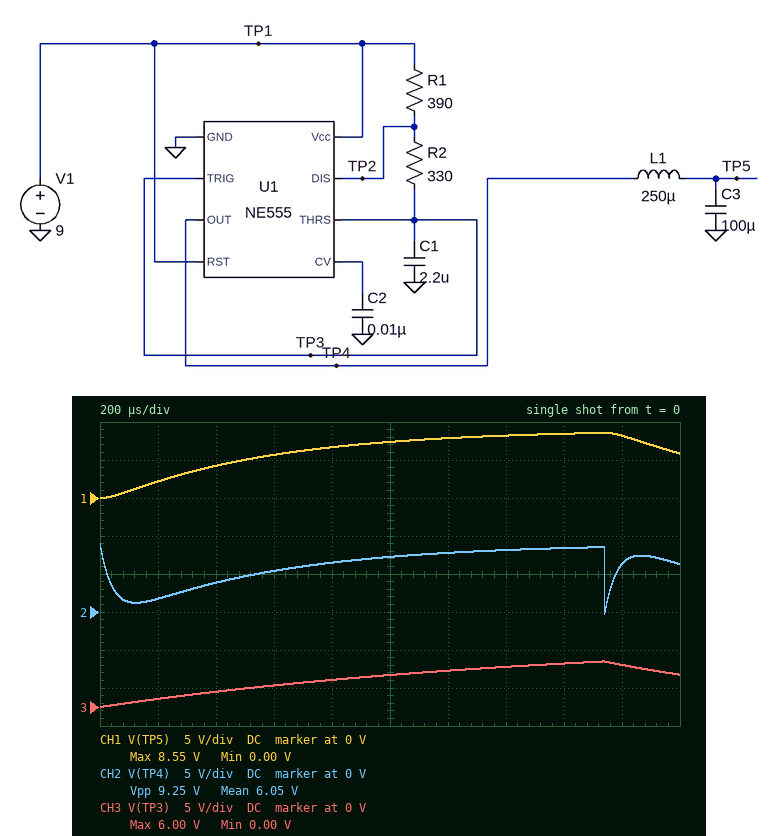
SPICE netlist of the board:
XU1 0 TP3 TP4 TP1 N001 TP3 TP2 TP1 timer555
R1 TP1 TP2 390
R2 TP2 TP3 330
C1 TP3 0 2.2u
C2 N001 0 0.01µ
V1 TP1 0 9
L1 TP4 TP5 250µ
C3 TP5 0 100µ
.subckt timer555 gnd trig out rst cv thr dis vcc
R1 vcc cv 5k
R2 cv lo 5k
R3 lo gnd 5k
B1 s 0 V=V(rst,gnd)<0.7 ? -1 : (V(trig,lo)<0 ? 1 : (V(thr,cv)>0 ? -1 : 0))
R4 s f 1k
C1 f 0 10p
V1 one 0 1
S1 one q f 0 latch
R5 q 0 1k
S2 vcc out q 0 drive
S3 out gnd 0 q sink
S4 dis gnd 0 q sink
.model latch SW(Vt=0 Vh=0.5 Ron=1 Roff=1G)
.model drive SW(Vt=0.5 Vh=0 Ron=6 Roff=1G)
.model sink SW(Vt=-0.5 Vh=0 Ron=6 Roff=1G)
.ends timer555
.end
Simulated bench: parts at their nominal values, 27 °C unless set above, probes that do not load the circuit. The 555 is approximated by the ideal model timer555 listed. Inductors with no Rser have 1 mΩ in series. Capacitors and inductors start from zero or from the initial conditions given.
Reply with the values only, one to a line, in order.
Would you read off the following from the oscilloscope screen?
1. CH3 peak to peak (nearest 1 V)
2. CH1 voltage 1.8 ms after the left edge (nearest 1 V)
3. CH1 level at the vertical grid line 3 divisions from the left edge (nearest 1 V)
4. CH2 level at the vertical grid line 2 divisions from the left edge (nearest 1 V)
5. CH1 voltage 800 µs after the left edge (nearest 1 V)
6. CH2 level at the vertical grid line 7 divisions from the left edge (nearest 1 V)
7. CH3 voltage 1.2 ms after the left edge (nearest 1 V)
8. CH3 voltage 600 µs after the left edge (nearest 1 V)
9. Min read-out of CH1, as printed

6 V
8 V
6 V
4 V
7 V
8 V
5 V
3 V
0.00 V
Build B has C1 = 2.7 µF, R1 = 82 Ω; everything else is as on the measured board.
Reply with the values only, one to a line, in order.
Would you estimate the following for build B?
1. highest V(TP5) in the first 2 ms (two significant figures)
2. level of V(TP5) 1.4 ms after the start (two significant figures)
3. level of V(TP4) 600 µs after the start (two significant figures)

7.9 V
6.3 V
5.4 V
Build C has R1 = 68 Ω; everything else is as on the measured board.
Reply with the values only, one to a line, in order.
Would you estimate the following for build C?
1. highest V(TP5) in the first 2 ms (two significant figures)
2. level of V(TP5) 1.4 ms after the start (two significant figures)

7.3 V
3.7 V
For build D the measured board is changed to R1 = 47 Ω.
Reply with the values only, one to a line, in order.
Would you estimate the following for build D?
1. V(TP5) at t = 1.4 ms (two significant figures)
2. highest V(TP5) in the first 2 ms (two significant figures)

3.3 V
7.1 V
